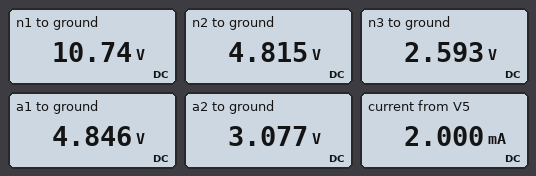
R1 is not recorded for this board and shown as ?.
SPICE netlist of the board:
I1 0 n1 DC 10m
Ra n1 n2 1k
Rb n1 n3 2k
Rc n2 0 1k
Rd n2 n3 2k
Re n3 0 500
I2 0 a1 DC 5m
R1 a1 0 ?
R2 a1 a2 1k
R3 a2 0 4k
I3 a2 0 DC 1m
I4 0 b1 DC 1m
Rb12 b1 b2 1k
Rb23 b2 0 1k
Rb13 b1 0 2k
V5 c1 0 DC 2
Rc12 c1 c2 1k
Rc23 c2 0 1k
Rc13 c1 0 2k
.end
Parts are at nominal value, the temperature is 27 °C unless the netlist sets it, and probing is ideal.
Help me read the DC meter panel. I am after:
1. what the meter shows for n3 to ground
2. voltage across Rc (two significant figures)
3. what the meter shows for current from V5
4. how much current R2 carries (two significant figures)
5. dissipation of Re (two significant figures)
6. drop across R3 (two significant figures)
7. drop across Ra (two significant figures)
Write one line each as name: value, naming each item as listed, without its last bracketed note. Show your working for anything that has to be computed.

what the meter shows for n3 to ground: 2.593 V
voltage across Rc: 4.815 V = 4.8 V
what the meter shows for current from V5: 2.000 mA
how much current R2 carries: (4.846 V - 3.077 V) / 1 kΩ = 1.8 mA
dissipation of Re: (2.593 V)^2 / 500 Ω = 13 mW
drop across R3: 3.077 V = 3.1 V
drop across Ra: 10.74 V - 4.815 V = 5.9 V
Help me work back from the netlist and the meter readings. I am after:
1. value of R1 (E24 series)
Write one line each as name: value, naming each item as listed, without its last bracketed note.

value of R1: 1.5 kΩ
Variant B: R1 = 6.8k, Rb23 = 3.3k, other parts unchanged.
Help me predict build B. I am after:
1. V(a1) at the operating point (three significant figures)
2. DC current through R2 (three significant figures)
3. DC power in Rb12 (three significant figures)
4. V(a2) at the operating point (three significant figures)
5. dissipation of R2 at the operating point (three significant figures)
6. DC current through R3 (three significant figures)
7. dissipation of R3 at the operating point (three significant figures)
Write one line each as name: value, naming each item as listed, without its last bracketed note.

V(a1) at the operating point: 12.1 V
DC current through R2: 3.22 mA
DC power in Rb12: 101 µW
V(a2) at the operating point: 8.88 V
dissipation of R2 at the operating point: 10.4 mW
DC current through R3: 2.22 mA
dissipation of R3 at the operating point: 19.7 mW
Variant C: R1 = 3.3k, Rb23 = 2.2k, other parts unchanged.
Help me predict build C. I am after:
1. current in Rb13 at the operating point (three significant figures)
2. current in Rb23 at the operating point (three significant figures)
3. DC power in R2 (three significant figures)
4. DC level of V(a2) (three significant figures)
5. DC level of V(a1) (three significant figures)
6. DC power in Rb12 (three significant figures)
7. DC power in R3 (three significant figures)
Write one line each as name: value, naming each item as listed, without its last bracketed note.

current in Rb13 at the operating point: 615 µA
current in Rb23 at the operating point: 385 µA
DC power in R2: 6.10 mW
DC level of V(a2): 5.88 V
DC level of V(a1): 8.35 V
DC power in Rb12: 148 µW
DC power in R3: 8.64 mW
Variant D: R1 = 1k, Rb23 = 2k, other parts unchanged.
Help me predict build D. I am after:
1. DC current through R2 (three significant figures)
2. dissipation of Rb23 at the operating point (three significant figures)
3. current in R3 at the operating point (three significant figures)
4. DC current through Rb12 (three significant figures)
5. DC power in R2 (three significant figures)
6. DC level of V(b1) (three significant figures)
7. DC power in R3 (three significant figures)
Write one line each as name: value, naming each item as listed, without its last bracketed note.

DC current through R2: 1.50 mA
dissipation of Rb23 at the operating point: 320 µW
current in R3 at the operating point: 500 µA
DC current through Rb12: 400 µA
DC power in R2: 2.25 mW
DC level of V(b1): 1.20 V
DC power in R3: 1.00 mW
